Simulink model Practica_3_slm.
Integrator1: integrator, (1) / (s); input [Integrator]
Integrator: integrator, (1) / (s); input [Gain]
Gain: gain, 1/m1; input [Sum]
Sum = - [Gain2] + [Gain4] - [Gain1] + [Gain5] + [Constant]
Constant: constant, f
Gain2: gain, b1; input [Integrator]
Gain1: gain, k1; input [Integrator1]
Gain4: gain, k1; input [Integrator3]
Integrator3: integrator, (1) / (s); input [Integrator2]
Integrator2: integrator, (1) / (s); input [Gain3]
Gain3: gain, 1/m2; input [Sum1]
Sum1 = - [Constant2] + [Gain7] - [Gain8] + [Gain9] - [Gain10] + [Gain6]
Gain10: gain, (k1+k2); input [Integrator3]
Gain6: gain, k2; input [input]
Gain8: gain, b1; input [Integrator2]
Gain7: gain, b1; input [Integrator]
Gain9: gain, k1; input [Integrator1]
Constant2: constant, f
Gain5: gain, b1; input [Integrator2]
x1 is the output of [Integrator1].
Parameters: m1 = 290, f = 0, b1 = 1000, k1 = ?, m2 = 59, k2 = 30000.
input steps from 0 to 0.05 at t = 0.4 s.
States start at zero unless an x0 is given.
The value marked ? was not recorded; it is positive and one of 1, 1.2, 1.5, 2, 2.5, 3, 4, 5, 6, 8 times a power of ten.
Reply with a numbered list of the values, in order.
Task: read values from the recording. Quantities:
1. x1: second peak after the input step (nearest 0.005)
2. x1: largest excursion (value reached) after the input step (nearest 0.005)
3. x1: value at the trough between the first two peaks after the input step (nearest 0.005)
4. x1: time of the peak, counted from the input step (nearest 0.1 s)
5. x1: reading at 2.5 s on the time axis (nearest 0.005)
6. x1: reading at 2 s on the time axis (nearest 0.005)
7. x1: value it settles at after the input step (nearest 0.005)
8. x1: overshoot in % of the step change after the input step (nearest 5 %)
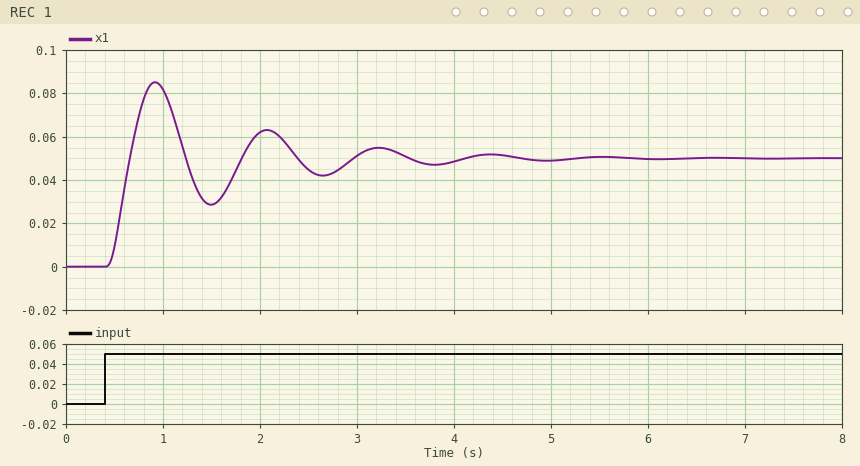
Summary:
1. 0.065
2. 0.085
3. 0.030
4. 0.5 s
5. 0.045
6. 0.060
7. 0.050
8. 70 %
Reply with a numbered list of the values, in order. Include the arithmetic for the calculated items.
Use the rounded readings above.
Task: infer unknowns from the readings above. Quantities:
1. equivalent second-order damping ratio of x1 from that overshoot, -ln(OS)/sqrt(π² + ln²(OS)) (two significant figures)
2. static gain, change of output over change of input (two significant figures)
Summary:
1. ln(0.7) = -0.357; 0.357 / sqrt(9.870 + 0.127) = 0.11
2. (0.05 - 0) / (0.05 - 0) = 1.0
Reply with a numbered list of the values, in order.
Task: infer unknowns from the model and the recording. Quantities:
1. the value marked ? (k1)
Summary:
1. 12000
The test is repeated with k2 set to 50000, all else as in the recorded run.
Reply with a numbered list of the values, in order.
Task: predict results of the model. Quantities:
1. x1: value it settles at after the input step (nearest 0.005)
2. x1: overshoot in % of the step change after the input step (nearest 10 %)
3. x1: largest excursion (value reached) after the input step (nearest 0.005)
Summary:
1. 0.050
2. 60 %
3. 0.080
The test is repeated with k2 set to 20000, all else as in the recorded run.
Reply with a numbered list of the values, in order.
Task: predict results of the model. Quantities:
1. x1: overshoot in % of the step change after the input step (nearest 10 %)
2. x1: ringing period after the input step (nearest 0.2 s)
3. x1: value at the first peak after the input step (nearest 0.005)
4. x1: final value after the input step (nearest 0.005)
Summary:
1. 80 %
2. 1.2 s
3. 0.090
4. 0.050
